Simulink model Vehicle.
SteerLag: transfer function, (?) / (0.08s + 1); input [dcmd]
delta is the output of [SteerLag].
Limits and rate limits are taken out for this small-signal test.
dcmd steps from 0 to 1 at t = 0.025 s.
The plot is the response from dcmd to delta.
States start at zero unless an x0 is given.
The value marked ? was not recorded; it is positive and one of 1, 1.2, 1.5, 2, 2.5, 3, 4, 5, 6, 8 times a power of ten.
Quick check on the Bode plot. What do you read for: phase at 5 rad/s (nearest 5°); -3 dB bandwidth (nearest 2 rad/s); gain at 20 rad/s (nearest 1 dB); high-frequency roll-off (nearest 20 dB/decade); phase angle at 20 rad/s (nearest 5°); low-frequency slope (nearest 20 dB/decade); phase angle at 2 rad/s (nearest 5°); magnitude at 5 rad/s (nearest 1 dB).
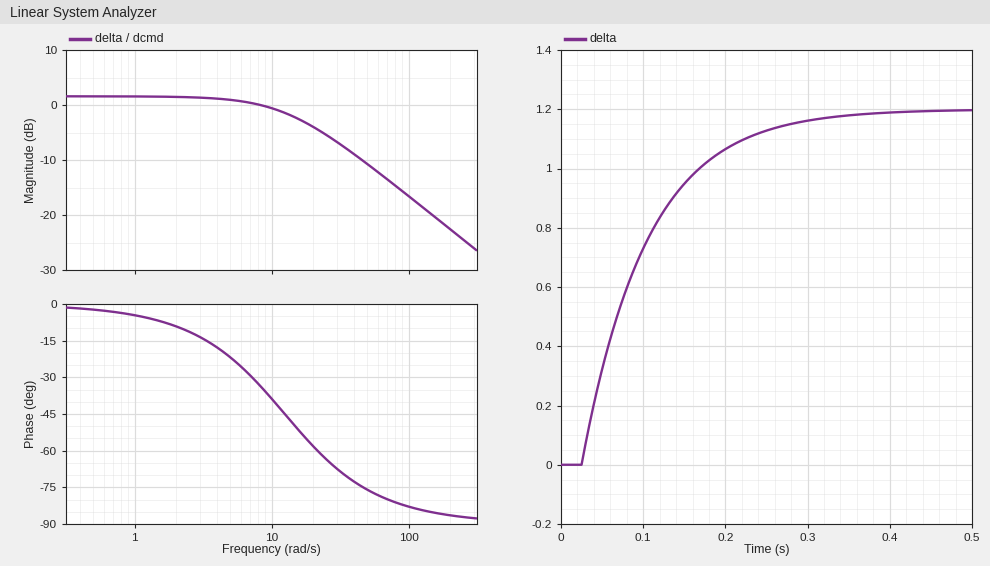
-20°
12 rad/s
-4 dB
-20 dB/decade
-60°
0 dB/decade
-10°
1 dB
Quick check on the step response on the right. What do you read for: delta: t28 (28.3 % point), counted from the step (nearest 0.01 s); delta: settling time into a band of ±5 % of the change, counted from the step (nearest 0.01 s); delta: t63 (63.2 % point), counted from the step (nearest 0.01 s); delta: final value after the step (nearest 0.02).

0.03 s
0.24 s
0.08 s
1.20
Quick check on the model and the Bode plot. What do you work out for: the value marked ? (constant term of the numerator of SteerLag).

1.2
